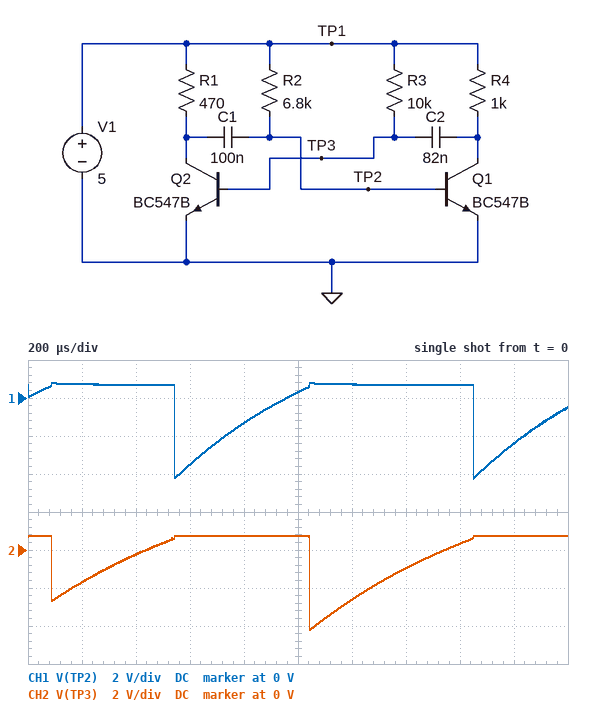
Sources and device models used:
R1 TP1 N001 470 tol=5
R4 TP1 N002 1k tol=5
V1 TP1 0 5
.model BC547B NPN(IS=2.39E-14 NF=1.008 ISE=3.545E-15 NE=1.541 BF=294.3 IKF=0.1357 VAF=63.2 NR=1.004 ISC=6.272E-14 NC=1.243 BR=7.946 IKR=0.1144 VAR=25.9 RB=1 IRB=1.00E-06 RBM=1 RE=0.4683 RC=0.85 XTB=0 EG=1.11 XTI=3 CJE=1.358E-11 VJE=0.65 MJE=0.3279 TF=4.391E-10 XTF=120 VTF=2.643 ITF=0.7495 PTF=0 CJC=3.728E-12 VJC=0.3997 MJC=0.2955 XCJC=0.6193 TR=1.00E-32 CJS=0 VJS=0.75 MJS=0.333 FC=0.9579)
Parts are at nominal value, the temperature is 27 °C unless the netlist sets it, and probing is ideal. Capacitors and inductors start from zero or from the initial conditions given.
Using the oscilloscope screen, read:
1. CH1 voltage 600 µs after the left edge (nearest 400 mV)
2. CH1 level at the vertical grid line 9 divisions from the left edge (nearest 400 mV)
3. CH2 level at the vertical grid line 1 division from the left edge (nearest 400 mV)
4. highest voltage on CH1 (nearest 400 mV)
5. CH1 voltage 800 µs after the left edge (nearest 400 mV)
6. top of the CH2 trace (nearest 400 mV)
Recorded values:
-3.6 V
-2.4 V
-1.6 V
800 mV
-1.2 V
800 mV
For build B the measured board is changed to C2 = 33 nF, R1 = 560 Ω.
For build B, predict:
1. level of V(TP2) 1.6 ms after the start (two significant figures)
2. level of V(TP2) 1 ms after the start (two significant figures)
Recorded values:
740 mV
710 mV
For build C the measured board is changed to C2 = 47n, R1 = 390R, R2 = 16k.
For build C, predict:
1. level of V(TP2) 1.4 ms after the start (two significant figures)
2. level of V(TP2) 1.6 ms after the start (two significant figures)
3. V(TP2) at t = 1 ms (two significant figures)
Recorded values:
-310 mV
310 mV
-1.8 V
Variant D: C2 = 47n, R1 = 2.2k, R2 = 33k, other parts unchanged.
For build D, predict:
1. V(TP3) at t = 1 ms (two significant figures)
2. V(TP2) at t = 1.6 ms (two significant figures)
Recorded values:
690 mV
-2.8 V
